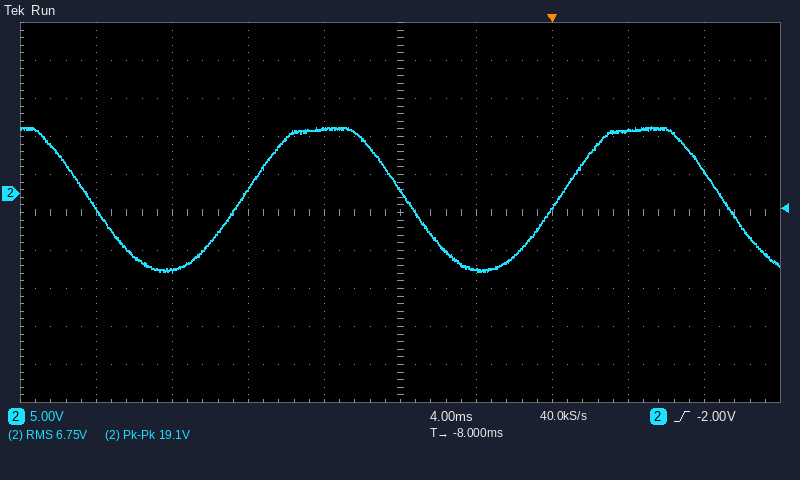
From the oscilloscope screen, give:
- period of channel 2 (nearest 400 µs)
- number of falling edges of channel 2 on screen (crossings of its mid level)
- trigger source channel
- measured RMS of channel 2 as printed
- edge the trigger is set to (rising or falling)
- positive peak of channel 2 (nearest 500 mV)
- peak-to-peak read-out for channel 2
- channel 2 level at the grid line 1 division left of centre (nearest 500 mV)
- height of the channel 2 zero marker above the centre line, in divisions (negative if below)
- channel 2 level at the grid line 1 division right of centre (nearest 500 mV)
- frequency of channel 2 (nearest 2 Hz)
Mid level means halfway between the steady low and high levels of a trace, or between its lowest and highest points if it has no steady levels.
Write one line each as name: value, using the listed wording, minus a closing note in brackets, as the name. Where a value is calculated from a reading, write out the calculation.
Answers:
period of channel 2: 16.8 ms
number of falling edges of channel 2 on screen: 3
trigger source channel: channel 2
measured RMS of channel 2 as printed: 6.75 V
edge the trigger is set to: rising
positive peak of channel 2: 9.0 V
peak-to-peak read-out for channel 2: 19.1 V
channel 2 level at the grid line 1 division left of centre: 8.5 V
height of the channel 2 zero marker above the centre line, in divisions: +0.5 div
channel 2 level at the grid line 1 division right of centre: -10.0 V
frequency of channel 2: 1 / 16.8 ms ≈ 60 Hz
